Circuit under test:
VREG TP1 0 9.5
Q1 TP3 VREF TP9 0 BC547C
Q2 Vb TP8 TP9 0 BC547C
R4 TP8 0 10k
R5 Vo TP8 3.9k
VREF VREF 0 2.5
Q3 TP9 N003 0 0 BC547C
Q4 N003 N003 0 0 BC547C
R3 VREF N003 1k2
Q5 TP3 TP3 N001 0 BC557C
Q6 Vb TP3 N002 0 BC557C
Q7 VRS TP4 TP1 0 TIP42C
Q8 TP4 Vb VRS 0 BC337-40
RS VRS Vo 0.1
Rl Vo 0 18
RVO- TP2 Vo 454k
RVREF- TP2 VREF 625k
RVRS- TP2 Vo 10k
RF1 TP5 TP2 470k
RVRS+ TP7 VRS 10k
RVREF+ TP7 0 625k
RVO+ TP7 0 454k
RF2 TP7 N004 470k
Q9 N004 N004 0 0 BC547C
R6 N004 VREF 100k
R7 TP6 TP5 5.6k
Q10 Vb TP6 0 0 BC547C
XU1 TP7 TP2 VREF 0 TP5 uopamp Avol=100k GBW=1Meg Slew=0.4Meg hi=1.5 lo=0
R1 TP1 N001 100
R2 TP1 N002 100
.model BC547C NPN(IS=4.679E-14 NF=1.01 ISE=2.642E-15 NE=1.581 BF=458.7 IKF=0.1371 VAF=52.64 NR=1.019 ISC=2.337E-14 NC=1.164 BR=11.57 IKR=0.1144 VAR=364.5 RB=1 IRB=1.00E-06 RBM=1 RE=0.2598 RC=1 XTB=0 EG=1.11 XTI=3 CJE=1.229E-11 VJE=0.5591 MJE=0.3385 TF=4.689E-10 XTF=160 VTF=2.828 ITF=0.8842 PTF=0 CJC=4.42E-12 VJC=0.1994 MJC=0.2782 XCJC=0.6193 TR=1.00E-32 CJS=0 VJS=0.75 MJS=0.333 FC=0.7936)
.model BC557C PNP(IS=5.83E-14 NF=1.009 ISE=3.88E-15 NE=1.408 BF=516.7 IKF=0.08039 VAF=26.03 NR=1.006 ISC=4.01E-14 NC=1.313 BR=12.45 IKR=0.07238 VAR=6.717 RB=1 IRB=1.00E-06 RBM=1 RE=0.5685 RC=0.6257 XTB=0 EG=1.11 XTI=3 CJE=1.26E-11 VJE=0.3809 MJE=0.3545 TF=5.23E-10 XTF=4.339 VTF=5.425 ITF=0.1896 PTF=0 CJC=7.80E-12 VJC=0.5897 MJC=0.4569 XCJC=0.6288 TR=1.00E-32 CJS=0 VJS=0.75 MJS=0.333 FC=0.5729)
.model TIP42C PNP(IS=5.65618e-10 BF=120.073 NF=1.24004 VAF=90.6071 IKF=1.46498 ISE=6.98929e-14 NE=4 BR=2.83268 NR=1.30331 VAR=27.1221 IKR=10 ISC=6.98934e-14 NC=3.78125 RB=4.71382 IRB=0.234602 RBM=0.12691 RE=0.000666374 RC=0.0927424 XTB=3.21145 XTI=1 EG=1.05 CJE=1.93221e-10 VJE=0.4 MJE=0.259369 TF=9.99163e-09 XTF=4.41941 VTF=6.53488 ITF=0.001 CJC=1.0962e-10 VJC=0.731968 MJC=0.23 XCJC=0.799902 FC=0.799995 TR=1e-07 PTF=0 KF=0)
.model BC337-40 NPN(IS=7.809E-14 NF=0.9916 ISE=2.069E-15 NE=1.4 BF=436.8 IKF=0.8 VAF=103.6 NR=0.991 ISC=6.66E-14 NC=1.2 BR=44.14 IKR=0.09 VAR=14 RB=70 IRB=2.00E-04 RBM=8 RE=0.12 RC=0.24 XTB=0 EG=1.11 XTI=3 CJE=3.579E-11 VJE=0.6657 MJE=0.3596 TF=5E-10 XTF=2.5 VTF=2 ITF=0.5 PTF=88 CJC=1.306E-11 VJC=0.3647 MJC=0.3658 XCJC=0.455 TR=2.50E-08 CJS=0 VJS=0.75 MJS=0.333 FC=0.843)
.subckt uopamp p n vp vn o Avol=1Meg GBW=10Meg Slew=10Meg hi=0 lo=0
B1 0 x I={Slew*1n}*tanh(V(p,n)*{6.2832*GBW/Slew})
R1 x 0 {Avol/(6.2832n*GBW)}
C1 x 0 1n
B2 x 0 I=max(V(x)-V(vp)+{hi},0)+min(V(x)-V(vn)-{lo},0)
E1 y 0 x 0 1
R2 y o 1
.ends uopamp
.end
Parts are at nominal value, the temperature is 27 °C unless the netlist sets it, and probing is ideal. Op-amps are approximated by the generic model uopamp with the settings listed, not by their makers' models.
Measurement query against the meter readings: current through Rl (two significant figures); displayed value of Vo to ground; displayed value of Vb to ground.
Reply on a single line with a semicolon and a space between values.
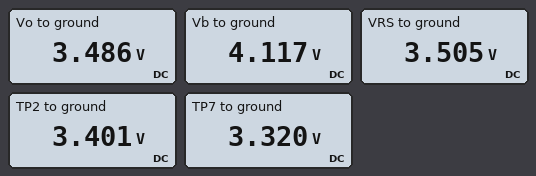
190 mA; 3.486 V; 4.117 V
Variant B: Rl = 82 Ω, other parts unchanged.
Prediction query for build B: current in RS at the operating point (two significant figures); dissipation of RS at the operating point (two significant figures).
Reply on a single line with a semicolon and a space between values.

43 mA; 180 µW
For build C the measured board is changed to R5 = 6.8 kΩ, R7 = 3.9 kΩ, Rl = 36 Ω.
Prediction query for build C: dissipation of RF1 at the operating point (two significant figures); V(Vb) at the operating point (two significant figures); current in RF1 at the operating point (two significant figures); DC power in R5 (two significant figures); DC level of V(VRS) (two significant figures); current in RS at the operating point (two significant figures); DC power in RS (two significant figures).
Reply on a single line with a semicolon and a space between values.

36 µW; 4.8 V; 8.7 µA; 430 µW; 4.2 V; 120 mA; 1.4 mW
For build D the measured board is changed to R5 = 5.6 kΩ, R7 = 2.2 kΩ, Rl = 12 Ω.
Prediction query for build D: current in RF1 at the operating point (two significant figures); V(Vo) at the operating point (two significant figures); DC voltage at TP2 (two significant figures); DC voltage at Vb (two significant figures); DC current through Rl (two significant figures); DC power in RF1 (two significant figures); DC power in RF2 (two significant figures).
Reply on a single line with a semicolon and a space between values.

8.1 µA; 3.9 V; 3.8 V; 4.6 V; 330 mA; 31 µW; 22 µW
